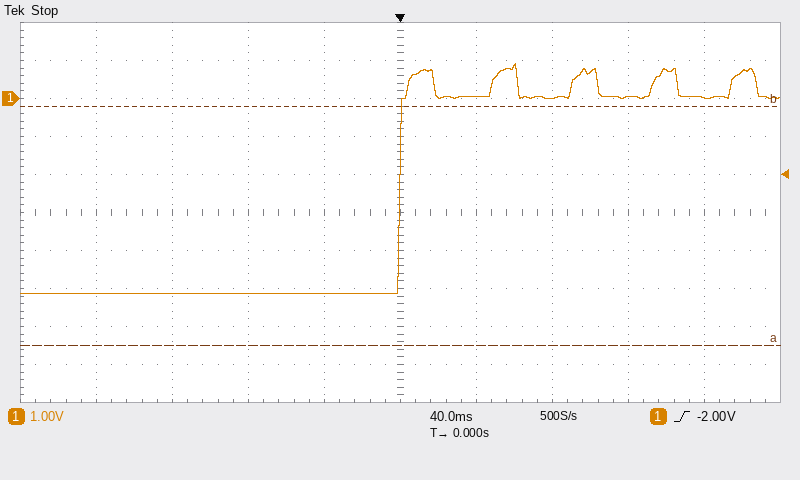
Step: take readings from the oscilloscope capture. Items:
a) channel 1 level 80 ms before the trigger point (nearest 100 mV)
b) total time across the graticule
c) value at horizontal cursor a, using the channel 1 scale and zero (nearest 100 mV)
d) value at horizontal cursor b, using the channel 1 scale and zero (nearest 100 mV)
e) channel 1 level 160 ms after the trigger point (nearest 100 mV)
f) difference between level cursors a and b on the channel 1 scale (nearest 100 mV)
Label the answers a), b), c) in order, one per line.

a) -5.1 V
b) 400 ms
c) -6.5 V
d) -200 mV
e) 0.0 V
f) 6.3 V
